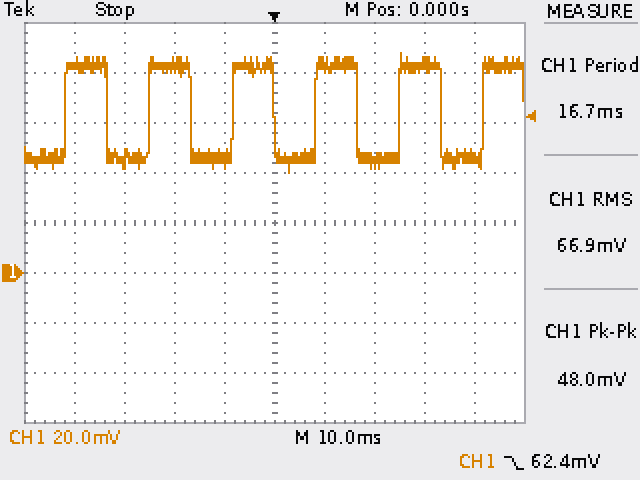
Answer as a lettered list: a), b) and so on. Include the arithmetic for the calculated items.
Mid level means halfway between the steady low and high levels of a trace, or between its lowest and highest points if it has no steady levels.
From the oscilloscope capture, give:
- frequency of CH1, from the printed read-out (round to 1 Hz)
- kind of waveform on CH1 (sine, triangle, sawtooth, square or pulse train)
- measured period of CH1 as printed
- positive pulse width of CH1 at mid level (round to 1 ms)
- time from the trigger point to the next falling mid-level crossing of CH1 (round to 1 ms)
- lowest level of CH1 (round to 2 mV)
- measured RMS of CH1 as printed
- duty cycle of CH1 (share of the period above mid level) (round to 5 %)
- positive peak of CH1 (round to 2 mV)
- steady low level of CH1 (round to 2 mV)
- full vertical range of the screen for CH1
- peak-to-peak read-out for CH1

a) 1 / 16.7 ms ≈ 60 Hz
b) square
c) 16.7 ms
d) 8 ms
e) 17 ms
f) 40 mV
g) 66.9 mV
h) 50 %
i) 88 mV
j) 46 mV
k) 160 mV
l) 48.0 mV
